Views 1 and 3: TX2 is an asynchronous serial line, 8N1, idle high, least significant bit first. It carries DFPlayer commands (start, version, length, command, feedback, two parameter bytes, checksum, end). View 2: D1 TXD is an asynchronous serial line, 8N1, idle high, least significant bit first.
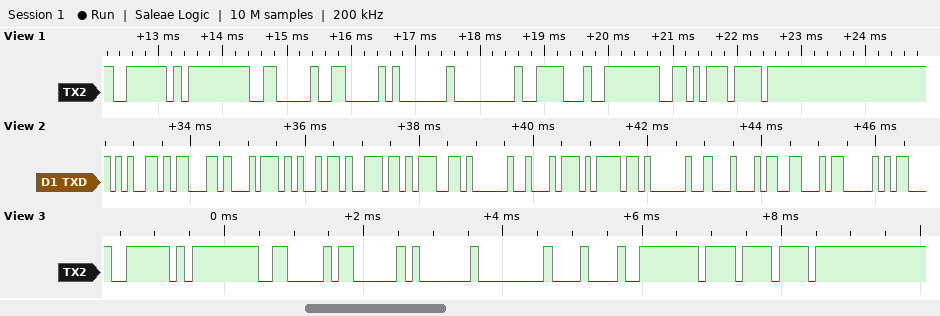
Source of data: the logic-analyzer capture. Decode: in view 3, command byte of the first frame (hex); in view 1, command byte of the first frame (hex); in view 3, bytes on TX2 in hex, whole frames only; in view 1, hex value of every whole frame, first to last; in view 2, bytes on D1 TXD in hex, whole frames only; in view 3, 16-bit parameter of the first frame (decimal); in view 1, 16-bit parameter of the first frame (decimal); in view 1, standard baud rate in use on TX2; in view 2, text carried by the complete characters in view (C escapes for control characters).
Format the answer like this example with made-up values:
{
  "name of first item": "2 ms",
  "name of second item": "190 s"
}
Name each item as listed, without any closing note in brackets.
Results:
{
  "in view 3, command byte of the first frame": "0x03",
  "in view 1, command byte of the first frame": "0x06",
  "in view 3, bytes on TX2 in hex, whole frames only": "7E FF 06 03 01 00 08 FE EF EF",
  "in view 1, hex value of every whole frame, first to last": "7E FF 06 06 01 00 1E FE D6 EF",
  "in view 2, bytes on D1 TXD in hex, whole frames only": "65 63 74 69 6E 67 20 74 6F 20 44 46 50",
  "in view 3, 16-bit parameter of the first frame": "8",
  "in view 1, 16-bit parameter of the first frame": "30",
  "in view 1, standard baud rate in use on TX2": "9600 baud",
  "in view 2, text carried by the complete characters in view": "\"ecting to DFP\""
}
